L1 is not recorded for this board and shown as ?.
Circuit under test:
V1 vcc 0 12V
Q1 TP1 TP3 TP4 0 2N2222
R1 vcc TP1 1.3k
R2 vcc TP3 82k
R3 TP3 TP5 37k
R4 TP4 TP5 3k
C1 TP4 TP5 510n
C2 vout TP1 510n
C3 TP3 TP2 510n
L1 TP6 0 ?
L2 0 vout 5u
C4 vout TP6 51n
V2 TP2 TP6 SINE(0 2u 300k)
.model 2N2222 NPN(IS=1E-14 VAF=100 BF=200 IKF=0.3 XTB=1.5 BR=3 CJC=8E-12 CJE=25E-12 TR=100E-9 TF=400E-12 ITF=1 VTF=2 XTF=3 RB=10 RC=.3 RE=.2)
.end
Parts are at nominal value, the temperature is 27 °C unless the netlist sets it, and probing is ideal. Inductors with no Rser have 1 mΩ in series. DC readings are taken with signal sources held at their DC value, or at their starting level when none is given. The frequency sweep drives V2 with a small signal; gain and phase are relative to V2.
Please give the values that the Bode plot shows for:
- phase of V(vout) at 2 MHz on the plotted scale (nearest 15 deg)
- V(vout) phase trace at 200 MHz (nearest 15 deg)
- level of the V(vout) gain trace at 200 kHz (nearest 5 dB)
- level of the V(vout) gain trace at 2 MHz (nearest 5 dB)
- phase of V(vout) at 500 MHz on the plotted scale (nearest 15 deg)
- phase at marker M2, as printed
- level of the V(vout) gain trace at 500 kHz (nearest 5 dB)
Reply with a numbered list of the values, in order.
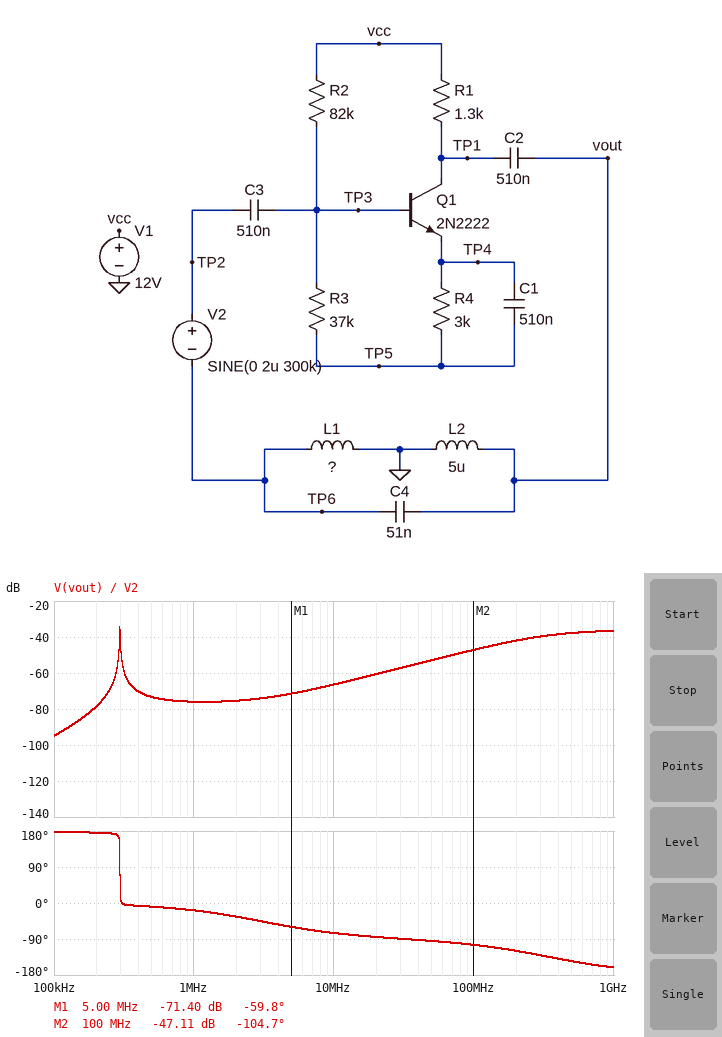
1. -30 deg
2. -120 deg
3. -80 dB
4. -75 dB
5. -150 deg
6. -104.7 deg
7. -75 dB
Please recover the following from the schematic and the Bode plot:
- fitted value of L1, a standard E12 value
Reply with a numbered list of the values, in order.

1. 680 nH
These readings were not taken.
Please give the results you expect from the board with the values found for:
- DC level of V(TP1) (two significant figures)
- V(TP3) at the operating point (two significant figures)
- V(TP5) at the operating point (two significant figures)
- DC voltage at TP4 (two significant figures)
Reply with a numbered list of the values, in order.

1. 12 V
2. 12 V
3. 12 V
4. 12 V
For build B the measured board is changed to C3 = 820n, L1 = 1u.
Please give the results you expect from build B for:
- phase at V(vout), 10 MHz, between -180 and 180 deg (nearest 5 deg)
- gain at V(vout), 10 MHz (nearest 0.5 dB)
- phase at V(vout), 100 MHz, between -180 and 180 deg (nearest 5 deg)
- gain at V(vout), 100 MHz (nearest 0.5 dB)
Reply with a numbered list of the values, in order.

1. -80 deg
2. -63.5 dB
3. -110 deg
4. -44.5 dB
